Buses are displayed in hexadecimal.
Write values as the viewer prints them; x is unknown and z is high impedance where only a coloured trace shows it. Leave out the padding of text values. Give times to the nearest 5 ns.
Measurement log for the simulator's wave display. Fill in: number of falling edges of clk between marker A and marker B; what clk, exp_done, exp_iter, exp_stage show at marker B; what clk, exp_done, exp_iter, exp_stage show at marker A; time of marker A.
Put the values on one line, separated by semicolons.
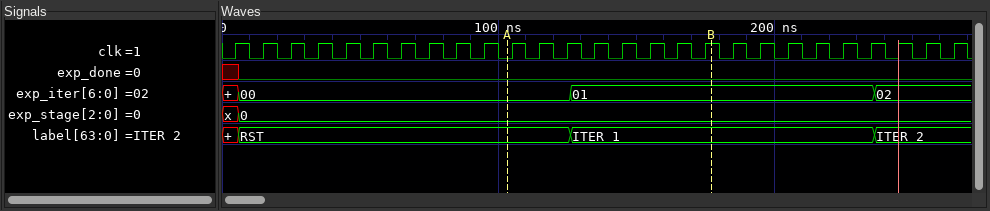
7; clk=1, exp_done=0, exp_iter=01, exp_stage=0; clk=0, exp_done=0, exp_iter=00, exp_stage=0; 105 ns
